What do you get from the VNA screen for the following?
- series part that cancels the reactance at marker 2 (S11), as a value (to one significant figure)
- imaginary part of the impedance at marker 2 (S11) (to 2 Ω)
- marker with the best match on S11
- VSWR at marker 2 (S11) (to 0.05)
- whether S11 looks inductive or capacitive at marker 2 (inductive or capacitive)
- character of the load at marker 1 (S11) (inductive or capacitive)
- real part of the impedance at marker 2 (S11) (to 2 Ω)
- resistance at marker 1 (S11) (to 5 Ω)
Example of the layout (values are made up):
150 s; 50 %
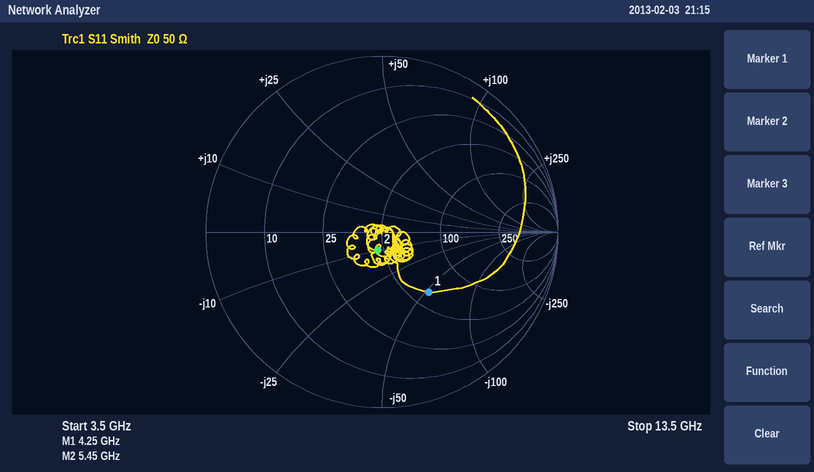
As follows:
300 pH; -10 Ω; marker 2; 1.25; capacitive; capacitive; 46 Ω; 60 Ω
